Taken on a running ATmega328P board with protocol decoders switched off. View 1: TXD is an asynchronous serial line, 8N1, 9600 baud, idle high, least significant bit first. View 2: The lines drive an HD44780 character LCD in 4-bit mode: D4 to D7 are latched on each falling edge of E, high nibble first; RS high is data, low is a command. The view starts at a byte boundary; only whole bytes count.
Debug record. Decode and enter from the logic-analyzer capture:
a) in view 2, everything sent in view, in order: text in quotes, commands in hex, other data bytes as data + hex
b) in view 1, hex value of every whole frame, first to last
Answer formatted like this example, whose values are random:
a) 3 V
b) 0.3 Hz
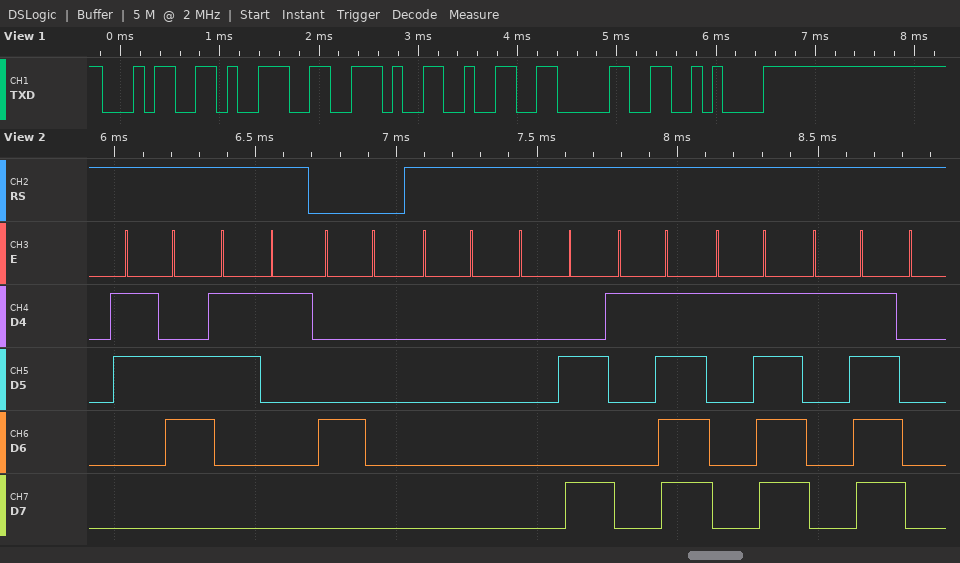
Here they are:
a) "61" 0x40 data 00 0A 1F 1F 1F
b) 34 39 2E 32 30 0A
